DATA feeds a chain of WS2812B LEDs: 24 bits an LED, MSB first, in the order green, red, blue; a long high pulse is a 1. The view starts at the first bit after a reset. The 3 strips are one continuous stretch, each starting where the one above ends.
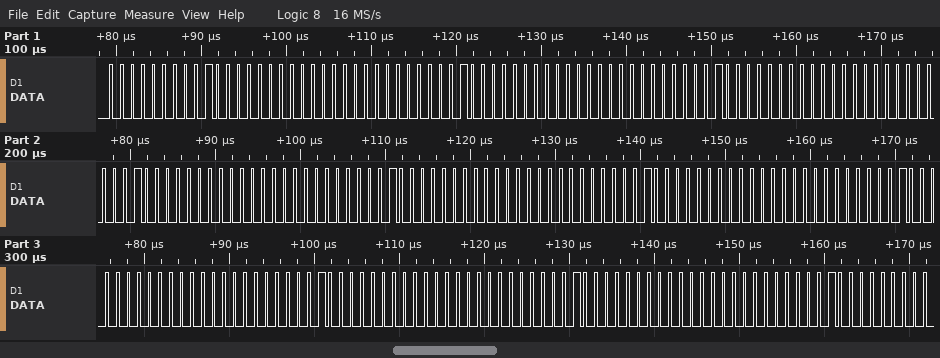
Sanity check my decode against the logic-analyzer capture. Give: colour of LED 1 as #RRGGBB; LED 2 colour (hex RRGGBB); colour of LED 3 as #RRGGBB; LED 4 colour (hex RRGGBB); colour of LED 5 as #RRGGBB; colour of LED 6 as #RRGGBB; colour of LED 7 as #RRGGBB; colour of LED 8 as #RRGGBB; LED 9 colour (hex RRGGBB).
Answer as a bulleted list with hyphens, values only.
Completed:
- #400000
- #400000
- #400000
- #400000
- #400000
- #400000
- #400000
- #400000
- #400000
